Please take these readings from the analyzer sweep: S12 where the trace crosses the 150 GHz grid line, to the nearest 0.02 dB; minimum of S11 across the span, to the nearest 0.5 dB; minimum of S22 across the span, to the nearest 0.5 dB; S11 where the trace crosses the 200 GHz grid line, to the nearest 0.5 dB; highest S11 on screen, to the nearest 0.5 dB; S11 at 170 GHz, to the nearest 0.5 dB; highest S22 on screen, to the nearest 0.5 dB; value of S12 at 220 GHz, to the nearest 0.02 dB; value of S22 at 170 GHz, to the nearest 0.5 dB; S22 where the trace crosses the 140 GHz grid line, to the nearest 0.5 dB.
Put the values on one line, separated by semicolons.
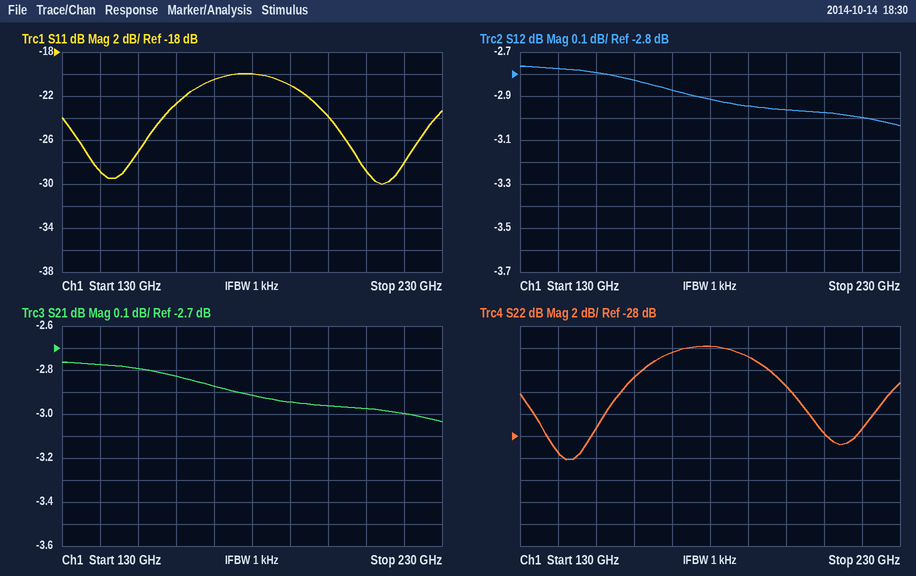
-2.80 dB; -30.0 dB; -30.0 dB; -24.0 dB; -20.0 dB; -20.5 dB; -20.0 dB; -3.00 dB; -20.5 dB; -29.5 dB
